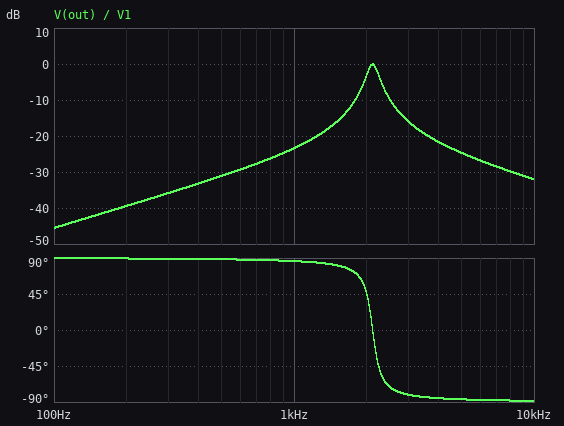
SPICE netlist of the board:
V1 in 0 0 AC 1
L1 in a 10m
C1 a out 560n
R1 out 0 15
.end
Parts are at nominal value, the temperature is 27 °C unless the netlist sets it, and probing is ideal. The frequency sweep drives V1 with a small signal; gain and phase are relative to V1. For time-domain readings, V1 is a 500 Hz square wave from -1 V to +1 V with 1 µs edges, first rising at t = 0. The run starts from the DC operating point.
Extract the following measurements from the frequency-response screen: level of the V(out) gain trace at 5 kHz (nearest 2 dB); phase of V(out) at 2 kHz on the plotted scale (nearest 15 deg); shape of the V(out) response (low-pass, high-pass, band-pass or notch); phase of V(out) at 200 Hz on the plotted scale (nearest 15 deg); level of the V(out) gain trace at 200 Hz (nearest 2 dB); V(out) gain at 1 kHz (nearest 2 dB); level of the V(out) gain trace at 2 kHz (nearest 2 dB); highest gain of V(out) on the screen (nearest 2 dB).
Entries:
-24 dB
45 deg
band-pass
90 deg
-40 dB
-24 dB
-4 dB
0 dB
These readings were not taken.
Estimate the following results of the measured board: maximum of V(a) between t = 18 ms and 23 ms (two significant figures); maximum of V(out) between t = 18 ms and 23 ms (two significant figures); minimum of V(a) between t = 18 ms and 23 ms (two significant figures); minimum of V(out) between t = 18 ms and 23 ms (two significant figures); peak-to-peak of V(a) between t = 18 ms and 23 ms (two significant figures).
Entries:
2.2 V
150 mV
-2.2 V
-150 mV
4.4 V
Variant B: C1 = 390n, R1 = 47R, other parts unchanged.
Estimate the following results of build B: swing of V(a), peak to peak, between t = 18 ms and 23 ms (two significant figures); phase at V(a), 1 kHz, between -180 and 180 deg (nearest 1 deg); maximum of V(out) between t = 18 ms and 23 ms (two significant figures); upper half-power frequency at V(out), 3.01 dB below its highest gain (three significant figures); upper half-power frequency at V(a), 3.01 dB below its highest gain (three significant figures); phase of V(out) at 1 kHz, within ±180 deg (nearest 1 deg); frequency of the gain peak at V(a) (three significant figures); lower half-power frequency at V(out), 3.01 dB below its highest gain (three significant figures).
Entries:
4.9 V
-1 deg
530 mV
2.95 kHz
2.85 kHz
82 deg
2.50 kHz
2.20 kHz
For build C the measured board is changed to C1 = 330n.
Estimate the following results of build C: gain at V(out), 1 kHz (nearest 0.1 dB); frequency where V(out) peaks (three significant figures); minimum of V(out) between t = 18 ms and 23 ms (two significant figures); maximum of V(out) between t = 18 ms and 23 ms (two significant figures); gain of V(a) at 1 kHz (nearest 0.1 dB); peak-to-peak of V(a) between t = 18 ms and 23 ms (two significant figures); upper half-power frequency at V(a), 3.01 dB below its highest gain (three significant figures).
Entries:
-28.9 dB
2.77 kHz
-140 mV
140 mV
1.2 dB
5.1 V
2.88 kHz
